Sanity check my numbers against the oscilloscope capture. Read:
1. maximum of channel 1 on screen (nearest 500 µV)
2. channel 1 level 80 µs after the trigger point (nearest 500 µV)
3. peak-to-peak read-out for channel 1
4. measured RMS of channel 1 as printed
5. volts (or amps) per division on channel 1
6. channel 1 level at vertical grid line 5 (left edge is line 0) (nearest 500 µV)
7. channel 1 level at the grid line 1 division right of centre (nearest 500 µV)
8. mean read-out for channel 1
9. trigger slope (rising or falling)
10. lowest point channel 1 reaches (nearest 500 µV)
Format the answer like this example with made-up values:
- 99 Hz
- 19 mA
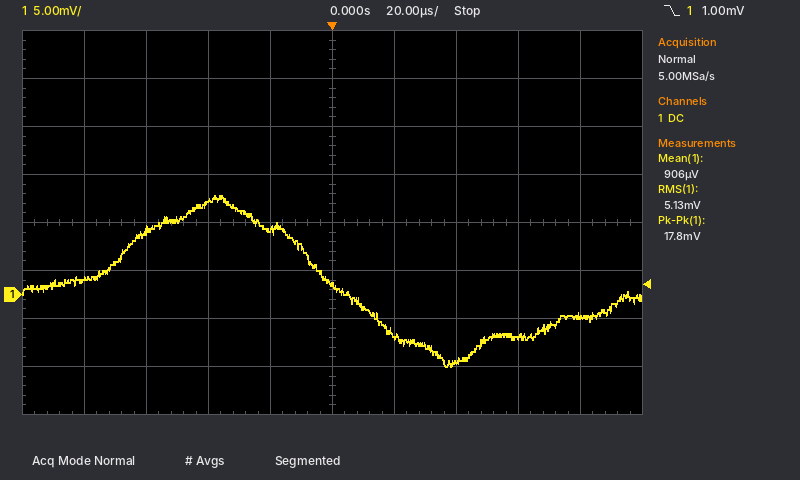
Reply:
- 10.5 mV
- -2.0 mV
- 17.8 mV
- 5.13 mV
- 5 mV
- 1.0 mV
- -4.5 mV
- 906 µV
- falling
- -7.5 mV
